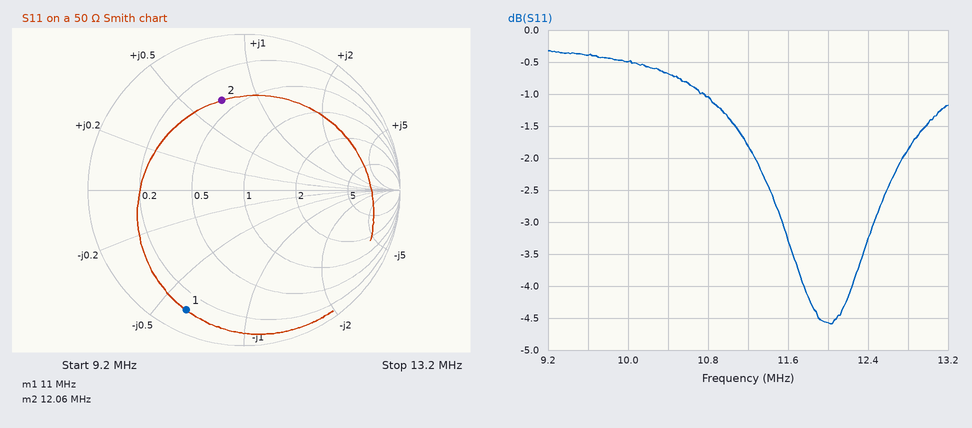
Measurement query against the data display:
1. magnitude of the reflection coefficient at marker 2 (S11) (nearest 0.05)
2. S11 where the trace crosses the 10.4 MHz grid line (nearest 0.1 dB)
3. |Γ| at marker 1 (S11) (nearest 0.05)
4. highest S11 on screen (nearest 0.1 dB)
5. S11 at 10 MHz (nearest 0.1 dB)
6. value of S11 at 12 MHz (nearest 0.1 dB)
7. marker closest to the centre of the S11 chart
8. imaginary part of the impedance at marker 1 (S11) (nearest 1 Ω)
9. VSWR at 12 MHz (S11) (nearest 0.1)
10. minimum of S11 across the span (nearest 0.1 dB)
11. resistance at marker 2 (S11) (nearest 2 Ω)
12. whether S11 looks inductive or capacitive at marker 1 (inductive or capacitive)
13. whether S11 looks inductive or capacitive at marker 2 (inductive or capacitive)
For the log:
0.60
-0.7 dB
0.85
-0.3 dB
-0.5 dB
-4.6 dB
marker 2
-31 Ω
3.9
-4.6 dB
20 Ω
capacitive
inductive
